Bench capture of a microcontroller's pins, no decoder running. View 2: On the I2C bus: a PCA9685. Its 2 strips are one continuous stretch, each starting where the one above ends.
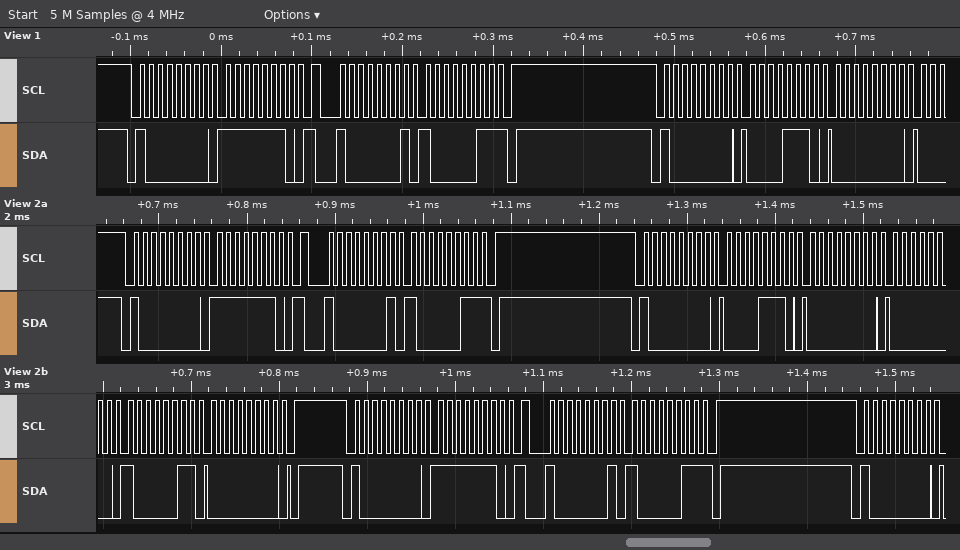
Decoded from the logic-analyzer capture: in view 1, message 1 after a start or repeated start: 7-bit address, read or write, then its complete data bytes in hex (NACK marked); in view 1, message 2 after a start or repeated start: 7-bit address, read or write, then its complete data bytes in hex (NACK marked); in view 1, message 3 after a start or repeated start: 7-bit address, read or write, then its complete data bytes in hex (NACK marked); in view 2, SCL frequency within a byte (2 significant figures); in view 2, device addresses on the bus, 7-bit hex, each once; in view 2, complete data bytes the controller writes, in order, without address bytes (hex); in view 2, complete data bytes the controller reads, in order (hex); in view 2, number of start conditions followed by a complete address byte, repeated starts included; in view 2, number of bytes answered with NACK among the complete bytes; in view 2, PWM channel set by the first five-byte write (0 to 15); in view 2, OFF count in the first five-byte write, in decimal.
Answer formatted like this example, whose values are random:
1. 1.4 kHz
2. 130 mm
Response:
1. 0x40 write: FE
2. 0x40 read: 83 NACK
3. 0x40 write: 0E 00
4. 100 kHz
5. 0x40
6. FE 0E 00 00 83 00 FE
7. 83 83
8. 6
9. 2
10. 2
11. 131
